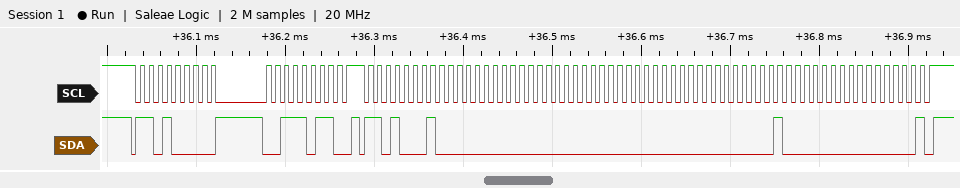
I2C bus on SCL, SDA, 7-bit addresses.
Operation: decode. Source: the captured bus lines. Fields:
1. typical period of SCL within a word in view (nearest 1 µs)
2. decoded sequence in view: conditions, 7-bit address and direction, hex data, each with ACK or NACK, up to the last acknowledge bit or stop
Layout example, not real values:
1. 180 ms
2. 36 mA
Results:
1. 10 µs
2. start, address 68 write ACK, 3B ACK, stop, start, address 68 read ACK, 00 ACK, 00 ACK, 00 ACK, 00 ACK, 40 ACK, 00 NACK, stop
